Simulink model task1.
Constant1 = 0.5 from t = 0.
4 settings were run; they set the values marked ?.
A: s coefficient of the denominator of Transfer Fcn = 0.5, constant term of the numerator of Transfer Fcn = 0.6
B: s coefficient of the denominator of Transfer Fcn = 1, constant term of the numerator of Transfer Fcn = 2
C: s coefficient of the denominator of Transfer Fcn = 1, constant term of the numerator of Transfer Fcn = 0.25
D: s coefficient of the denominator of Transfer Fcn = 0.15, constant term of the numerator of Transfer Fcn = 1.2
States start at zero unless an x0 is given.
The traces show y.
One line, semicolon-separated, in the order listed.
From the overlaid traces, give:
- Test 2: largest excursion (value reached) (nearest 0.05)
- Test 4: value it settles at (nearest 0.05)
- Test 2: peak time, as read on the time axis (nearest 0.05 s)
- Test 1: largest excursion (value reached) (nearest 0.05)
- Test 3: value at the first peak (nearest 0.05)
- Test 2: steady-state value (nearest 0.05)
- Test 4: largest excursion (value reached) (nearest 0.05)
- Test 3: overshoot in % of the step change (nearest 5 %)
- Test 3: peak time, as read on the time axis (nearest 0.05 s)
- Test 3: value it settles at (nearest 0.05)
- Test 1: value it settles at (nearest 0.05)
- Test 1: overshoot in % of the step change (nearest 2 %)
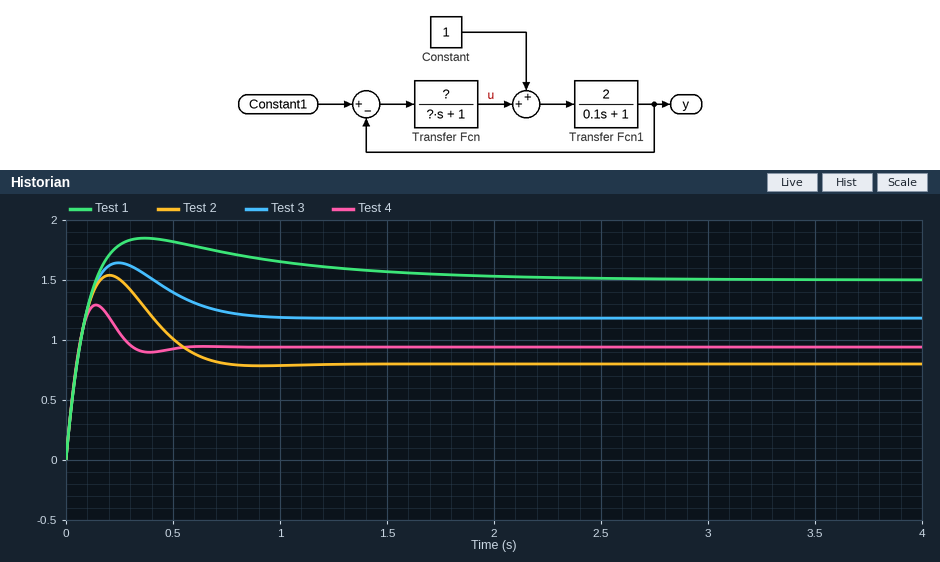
1.55; 0.95; 0.20 s; 1.85; 1.65; 0.80; 1.30; 40 %; 0.25 s; 1.20; 1.50; 24 %
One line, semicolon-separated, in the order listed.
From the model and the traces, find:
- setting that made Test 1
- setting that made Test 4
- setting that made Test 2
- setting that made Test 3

C; D; B; A
